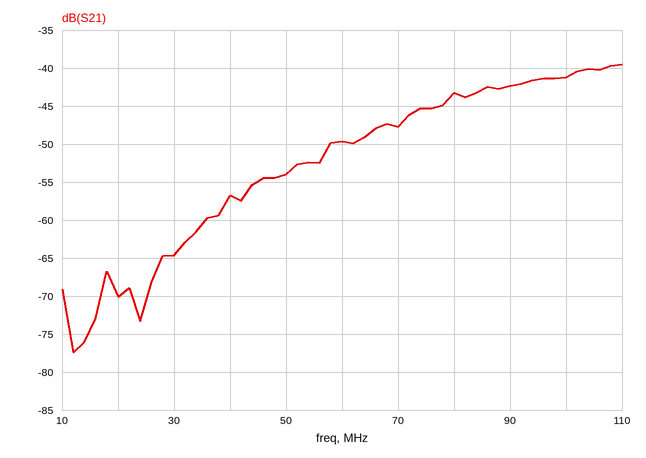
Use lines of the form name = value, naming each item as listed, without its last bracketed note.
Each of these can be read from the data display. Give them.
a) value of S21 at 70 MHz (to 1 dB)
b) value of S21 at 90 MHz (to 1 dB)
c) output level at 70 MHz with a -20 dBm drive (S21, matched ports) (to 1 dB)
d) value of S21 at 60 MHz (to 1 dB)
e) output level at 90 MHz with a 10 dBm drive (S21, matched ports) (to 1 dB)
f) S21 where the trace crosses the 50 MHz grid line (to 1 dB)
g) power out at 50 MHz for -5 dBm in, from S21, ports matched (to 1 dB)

value of S21 at 70 MHz = -48 dB
value of S21 at 90 MHz = -42 dB
output level at 70 MHz with a -20 dBm drive (S21, matched ports) = -68 dBm
value of S21 at 60 MHz = -50 dB
output level at 90 MHz with a 10 dBm drive (S21, matched ports) = -32 dBm
S21 where the trace crosses the 50 MHz grid line = -54 dB
power out at 50 MHz for -5 dBm in, from S21, ports matched = -59 dBm
